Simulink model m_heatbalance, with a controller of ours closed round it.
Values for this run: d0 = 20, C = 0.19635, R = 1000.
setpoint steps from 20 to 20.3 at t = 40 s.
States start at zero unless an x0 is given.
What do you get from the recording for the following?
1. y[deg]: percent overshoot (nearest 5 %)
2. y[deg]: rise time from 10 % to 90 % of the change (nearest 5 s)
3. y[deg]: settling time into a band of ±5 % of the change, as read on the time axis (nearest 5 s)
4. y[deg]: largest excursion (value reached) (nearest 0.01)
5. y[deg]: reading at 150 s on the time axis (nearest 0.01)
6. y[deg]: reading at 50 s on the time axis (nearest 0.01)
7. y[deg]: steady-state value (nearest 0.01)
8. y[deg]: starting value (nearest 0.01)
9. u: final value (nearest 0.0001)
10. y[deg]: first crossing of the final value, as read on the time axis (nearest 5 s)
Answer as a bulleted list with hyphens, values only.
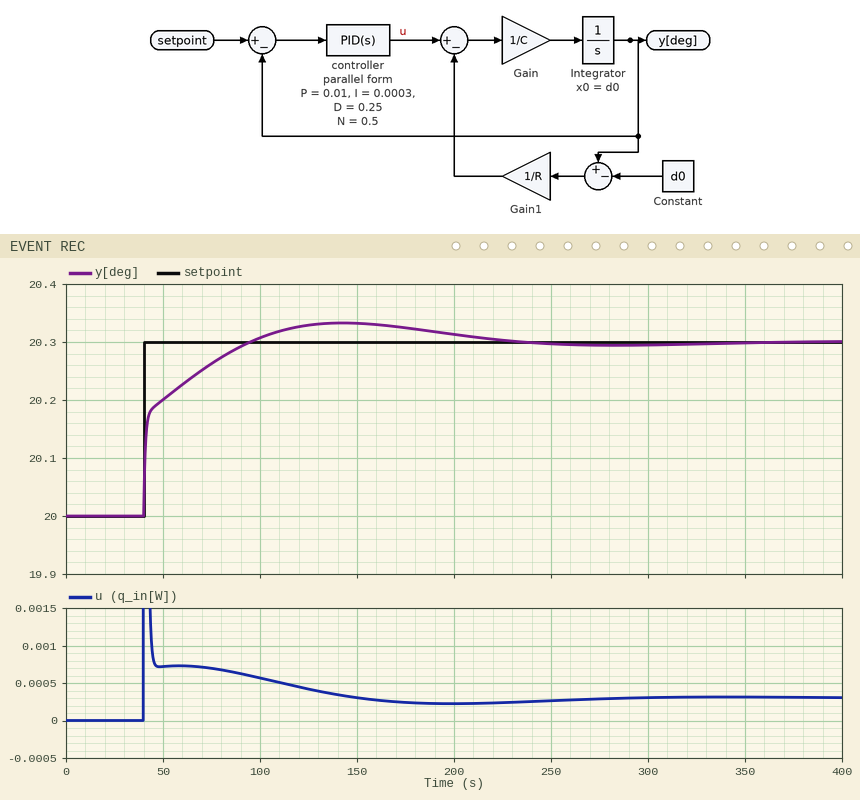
- 10 %
- 40 s
- 195 s
- 20.33
- 20.33
- 20.20
- 20.30
- 20.00
- 0.0003
- 95 s
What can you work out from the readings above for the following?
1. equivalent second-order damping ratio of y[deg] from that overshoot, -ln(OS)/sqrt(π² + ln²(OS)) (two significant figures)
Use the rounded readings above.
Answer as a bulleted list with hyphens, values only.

- 0.59
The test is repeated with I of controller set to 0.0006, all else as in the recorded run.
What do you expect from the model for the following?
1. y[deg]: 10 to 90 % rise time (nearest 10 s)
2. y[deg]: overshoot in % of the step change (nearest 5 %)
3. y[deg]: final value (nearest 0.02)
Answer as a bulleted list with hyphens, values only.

- 30 s
- 15 %
- 20.30
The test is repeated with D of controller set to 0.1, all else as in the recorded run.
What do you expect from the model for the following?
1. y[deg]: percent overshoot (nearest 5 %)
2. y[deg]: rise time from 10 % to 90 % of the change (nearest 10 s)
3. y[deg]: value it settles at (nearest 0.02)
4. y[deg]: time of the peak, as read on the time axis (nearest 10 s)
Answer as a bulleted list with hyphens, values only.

- 15 %
- 30 s
- 20.30
- 120 s
